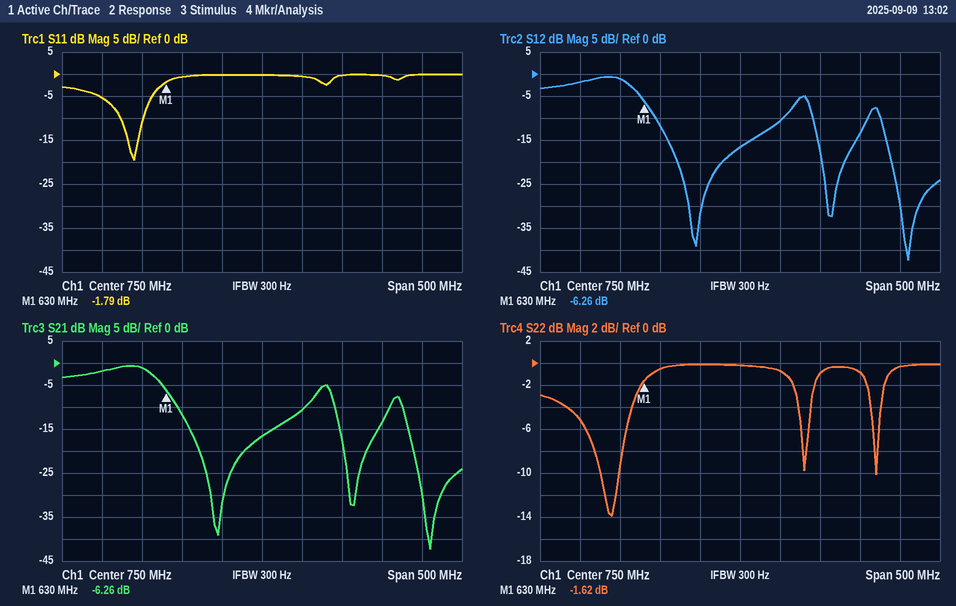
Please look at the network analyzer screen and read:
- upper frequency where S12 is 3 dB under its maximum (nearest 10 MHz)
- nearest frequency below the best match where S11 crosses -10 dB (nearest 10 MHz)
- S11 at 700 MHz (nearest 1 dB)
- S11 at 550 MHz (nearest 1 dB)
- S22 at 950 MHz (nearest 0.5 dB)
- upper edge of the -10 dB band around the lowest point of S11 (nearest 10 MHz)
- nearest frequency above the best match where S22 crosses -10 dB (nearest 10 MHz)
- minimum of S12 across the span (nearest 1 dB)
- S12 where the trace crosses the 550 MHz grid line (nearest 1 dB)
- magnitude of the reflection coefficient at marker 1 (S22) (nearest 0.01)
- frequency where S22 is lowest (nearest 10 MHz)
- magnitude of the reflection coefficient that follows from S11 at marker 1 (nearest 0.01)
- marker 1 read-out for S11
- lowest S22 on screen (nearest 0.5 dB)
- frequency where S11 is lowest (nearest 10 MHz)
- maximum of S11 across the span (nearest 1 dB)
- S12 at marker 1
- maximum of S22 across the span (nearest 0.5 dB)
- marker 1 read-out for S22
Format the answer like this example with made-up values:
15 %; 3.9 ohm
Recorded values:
620 MHz; 570 MHz; 0 dB; -5 dB; -0.5 dB; 600 MHz; 600 MHz; -42 dB; -2 dB; 0.83; 590 MHz; 0.81; -1.79 dB; -14.0 dB; 590 MHz; 0 dB; -6.26 dB; 0.0 dB; -1.62 dB
